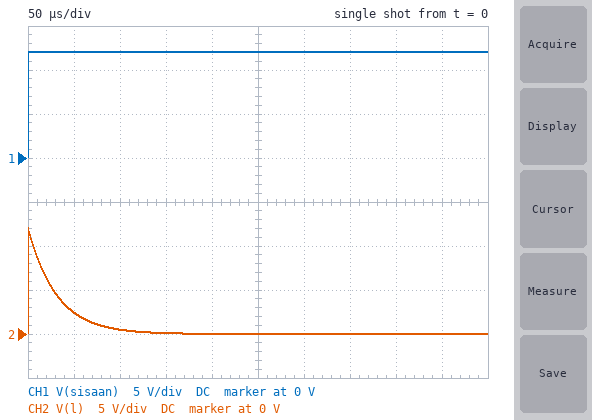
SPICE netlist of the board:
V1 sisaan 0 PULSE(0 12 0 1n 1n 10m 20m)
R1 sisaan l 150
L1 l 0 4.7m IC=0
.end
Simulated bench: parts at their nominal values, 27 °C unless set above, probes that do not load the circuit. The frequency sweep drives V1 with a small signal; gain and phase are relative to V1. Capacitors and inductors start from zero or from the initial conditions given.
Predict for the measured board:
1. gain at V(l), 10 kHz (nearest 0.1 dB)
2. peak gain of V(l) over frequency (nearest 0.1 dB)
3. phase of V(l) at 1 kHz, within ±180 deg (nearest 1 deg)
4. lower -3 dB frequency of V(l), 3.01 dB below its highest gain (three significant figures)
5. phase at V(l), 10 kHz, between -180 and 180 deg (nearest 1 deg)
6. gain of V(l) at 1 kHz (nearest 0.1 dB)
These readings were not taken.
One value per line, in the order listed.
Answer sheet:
-1.0 dB
0 dB
79 deg
5.08 kHz
27 deg
-14.3 dB
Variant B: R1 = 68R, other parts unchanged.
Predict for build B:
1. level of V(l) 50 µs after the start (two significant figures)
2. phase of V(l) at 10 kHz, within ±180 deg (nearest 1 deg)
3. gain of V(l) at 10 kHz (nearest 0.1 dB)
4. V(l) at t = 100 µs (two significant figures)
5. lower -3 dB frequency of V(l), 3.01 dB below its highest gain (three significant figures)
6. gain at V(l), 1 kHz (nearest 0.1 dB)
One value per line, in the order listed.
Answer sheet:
5.8 V
13 deg
-0.2 dB
2.8 V
2.30 kHz
-8.0 dB
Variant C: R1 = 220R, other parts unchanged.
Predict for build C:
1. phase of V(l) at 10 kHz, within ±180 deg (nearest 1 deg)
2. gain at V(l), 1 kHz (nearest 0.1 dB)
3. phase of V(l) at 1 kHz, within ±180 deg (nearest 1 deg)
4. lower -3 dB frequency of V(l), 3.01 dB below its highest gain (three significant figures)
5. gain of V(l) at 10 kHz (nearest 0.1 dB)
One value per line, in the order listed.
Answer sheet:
37 deg
-17.5 dB
82 deg
7.45 kHz
-1.9 dB
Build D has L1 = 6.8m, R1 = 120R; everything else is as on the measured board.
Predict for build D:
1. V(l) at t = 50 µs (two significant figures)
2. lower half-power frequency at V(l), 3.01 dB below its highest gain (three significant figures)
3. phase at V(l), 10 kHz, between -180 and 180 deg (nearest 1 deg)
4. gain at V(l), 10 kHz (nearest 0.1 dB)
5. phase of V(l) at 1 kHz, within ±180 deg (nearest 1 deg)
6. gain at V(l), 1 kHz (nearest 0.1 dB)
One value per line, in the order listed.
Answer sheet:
5.0 V
2.81 kHz
16 deg
-0.3 dB
70 deg
-9.5 dB
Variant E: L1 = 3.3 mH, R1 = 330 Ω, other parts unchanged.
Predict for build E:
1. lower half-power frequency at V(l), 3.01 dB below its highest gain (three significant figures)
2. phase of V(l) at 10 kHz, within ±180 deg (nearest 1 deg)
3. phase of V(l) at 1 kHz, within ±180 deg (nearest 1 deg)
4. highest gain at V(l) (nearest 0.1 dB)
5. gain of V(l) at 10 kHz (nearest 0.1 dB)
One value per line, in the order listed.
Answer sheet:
15.9 kHz
58 deg
86 deg
0 dB
-5.5 dB
